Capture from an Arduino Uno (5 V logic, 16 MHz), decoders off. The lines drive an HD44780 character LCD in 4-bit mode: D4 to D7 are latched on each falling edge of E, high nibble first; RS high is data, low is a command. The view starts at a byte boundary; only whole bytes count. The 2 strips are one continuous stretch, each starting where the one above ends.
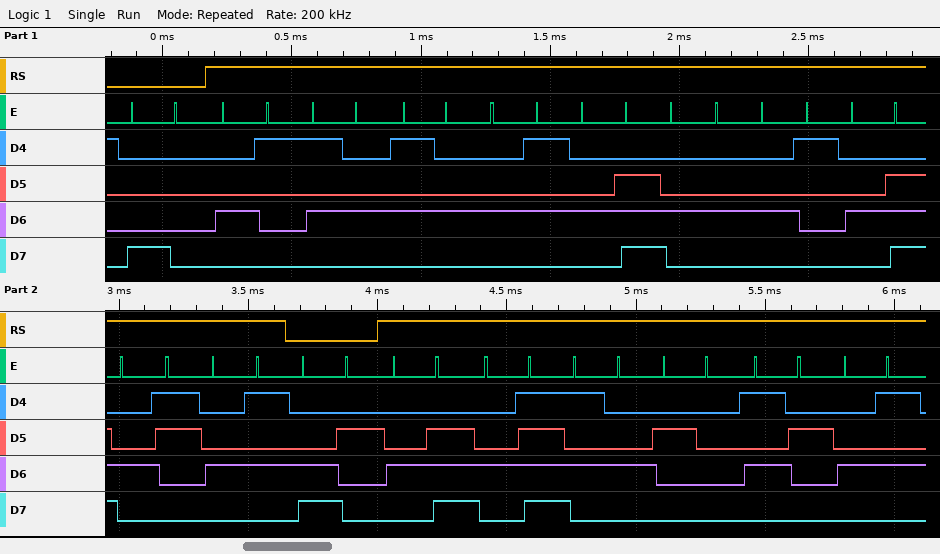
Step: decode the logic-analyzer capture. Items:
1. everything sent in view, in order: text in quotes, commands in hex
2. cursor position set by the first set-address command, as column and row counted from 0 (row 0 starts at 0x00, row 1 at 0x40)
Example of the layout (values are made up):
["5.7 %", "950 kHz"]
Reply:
["0x80 \"ATTENDANCE\" 0xC2 \"NOT RE\"", "column 0, row 0"]
